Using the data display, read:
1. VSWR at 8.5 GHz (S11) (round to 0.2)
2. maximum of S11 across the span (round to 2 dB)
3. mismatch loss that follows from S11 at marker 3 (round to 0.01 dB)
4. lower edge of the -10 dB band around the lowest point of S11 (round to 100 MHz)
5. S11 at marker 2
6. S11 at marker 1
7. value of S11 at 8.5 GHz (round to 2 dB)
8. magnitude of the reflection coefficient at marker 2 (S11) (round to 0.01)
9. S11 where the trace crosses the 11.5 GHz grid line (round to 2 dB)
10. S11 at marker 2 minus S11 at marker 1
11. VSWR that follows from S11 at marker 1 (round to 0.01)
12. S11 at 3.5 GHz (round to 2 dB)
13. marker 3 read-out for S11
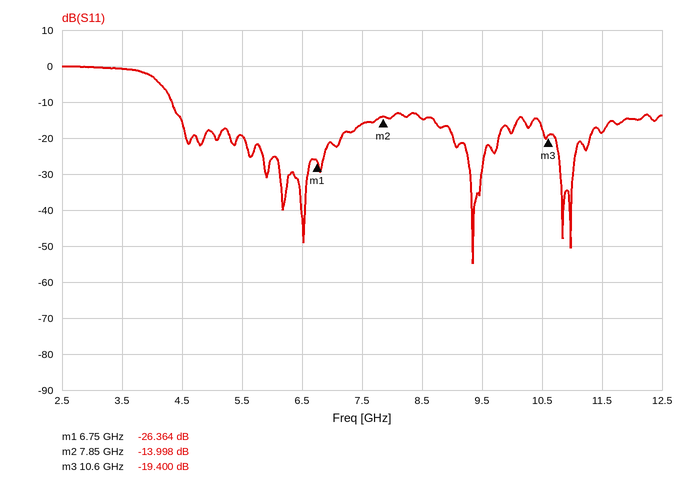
1.4
0 dB
0.05 dB
4.3 GHz
-13.998 dB
-26.364 dB
-14 dB
0.20
-18 dB
12.366 dB
1.10
0 dB
-19.400 dB
